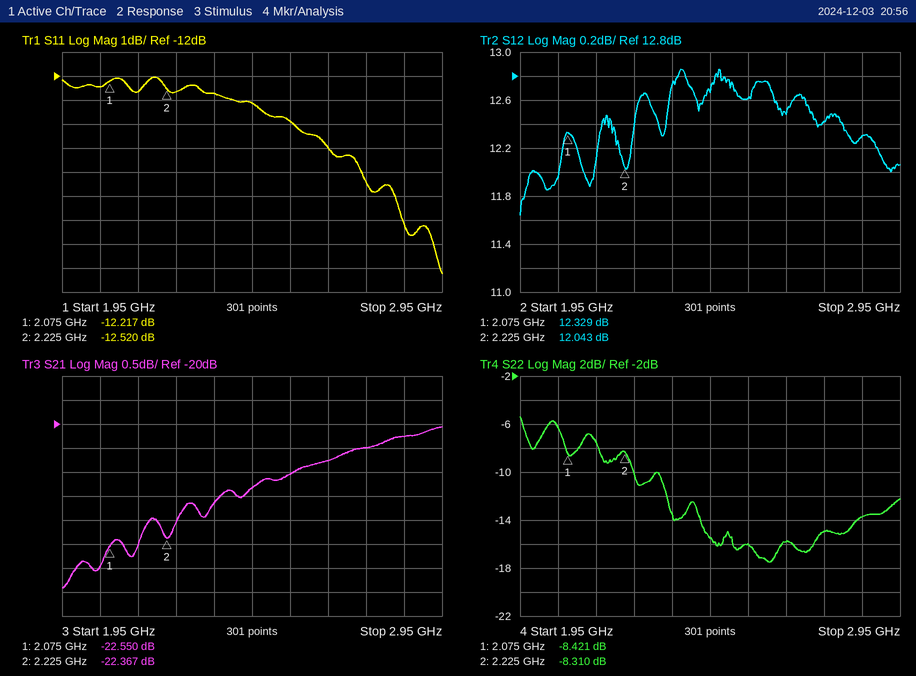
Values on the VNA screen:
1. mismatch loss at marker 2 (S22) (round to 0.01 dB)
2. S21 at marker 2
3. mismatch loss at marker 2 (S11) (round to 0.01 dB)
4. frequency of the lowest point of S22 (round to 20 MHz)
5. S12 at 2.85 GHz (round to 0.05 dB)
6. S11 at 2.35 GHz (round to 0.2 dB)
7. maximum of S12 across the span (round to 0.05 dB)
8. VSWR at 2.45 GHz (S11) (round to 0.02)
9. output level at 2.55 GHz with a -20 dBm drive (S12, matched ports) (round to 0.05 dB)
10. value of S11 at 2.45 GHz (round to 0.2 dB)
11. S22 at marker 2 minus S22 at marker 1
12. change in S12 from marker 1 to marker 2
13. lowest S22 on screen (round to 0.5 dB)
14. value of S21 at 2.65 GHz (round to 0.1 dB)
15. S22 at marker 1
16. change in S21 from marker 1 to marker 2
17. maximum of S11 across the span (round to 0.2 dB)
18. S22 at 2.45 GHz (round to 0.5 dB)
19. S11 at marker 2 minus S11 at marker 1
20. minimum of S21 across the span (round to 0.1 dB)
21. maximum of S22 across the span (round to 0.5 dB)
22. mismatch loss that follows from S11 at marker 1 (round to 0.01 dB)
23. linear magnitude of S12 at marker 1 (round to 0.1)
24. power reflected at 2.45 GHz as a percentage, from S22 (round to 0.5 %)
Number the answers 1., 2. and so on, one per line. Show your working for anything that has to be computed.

1. −10 log10(1 − 10^(-8.31/10)) ≈ 0.69 dB
2. -22.367 dB
3. −10 log10(1 − 10^(-12.52/10)) ≈ 0.25 dB
4. 2.60 GHz
5. 12.30 dB
6. -12.8 dB
7. 12.85 dB
8. |Γ| = 10^(-13.2/20) = 0.2188; VSWR = (1 + 0.2188)/(1 − 0.2188) ≈ 1.56
9. -20 dBm + (12.60 dB) = -7.40 dBm
10. -13.2 dB
11. -8.31 − (-8.421) = 0.111 dB
12. 12.043 − (12.329) = -0.286 dB
13. -17.5 dB
14. -20.8 dB
15. -8.421 dB
16. -22.367 − (-22.55) = 0.183 dB
17. -12.0 dB
18. -15.5 dB
19. -12.52 − (-12.217) = -0.303 dB
20. -23.4 dB
21. -5.5 dB
22. −10 log10(1 − 10^(-12.217/10)) ≈ 0.27 dB
23. 10^(12.329/20) ≈ 4.1
24. 10^(-15.5/10) ≈ 2.82 %, so 3.0 % to the nearest 0.5 %
